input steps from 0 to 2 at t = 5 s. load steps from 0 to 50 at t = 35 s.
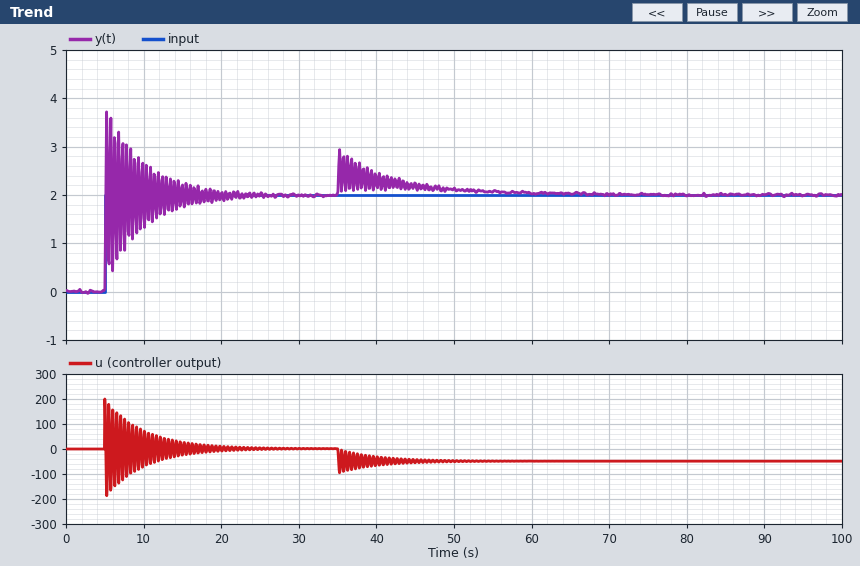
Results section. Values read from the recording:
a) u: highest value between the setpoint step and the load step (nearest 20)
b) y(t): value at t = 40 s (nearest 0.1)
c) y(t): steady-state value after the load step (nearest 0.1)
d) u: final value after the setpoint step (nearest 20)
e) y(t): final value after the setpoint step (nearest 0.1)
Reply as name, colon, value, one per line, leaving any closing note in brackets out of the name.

u: highest value between the setpoint step and the load step: 200
y(t): value at t = 40 s: 2.3
y(t): steady-state value after the load step: 2.0
u: final value after the setpoint step: 0
y(t): final value after the setpoint step: 2.0
